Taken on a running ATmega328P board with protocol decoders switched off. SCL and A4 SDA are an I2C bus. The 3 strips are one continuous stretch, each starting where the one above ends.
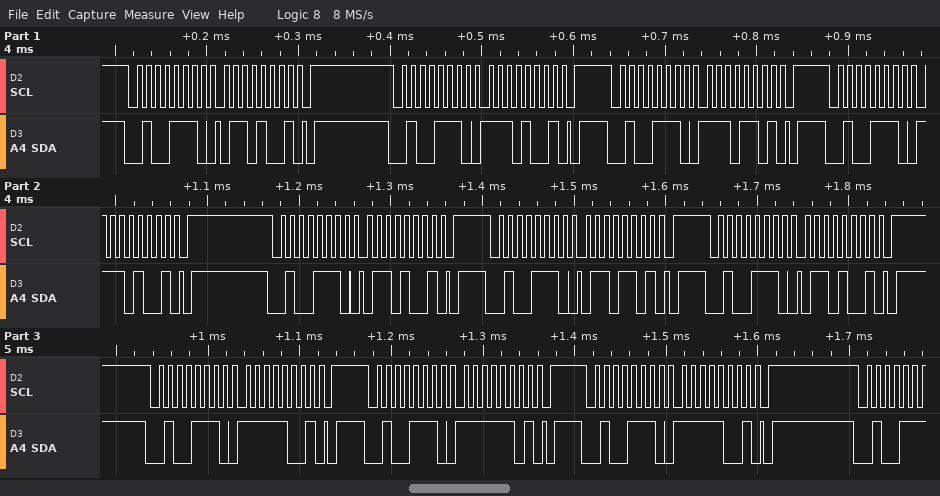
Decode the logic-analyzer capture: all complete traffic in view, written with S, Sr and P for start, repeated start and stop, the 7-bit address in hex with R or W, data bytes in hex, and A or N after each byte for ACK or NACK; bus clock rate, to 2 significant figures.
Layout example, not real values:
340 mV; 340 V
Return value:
S 27W A 69 A P S 27W A E9 A P S 27W A ED A P S 27W A E9 A P S 27W A 69 A P S 27W A 6D A P S 27W A 69 A P S 27W A F9 A P S 27W A FD A P S 27W A F9 A P; 100 kHz
